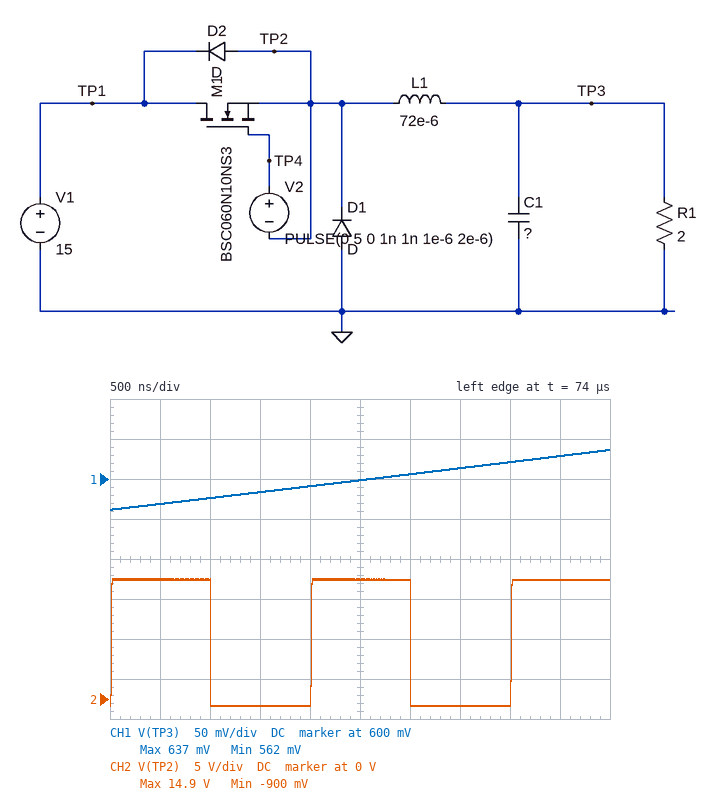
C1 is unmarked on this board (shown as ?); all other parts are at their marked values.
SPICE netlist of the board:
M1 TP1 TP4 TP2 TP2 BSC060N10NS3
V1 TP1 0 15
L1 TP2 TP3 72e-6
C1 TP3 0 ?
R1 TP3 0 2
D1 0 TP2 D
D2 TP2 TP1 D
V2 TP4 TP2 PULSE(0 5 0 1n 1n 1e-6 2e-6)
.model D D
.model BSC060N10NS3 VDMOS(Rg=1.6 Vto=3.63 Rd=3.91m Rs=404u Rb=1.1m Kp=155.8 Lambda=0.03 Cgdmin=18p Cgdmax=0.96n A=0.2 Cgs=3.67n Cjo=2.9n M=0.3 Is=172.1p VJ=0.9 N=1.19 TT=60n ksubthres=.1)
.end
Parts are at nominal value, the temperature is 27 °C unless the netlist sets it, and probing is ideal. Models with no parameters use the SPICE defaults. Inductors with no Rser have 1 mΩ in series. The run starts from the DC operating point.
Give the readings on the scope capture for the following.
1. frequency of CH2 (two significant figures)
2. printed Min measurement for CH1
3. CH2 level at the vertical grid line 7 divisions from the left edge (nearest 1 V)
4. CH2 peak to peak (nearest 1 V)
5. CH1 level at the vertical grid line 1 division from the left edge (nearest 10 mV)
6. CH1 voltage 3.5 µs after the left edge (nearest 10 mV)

500 kHz
562 mV
-1 V
16 V
570 mV
610 mV
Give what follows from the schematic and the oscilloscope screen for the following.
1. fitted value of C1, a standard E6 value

470 µF
